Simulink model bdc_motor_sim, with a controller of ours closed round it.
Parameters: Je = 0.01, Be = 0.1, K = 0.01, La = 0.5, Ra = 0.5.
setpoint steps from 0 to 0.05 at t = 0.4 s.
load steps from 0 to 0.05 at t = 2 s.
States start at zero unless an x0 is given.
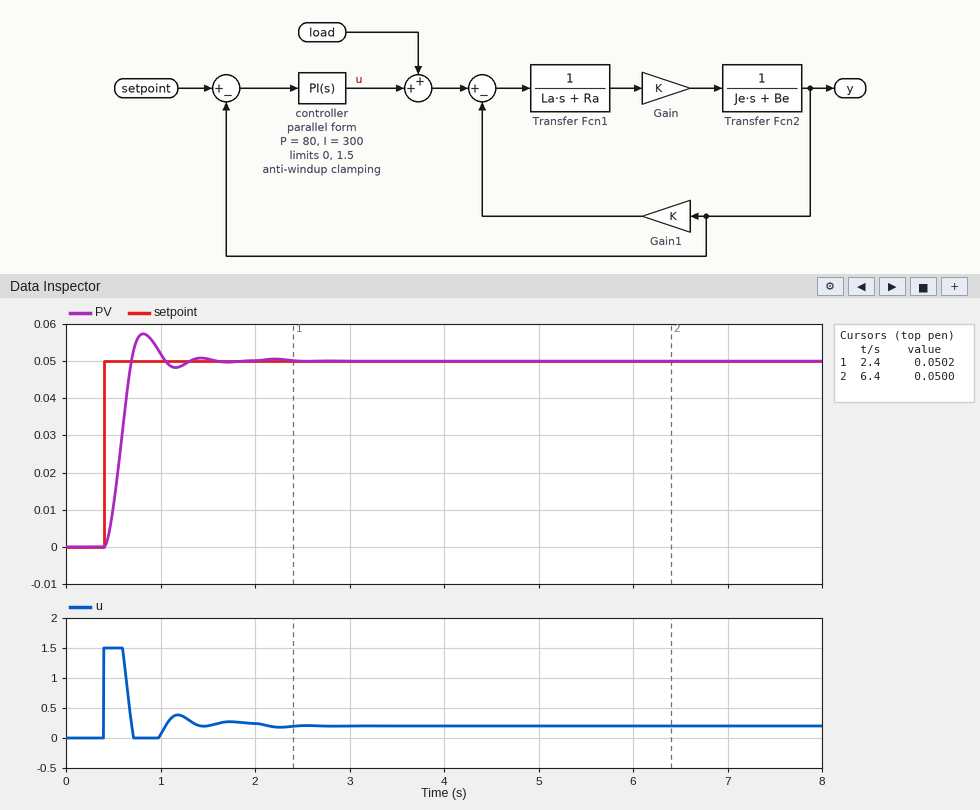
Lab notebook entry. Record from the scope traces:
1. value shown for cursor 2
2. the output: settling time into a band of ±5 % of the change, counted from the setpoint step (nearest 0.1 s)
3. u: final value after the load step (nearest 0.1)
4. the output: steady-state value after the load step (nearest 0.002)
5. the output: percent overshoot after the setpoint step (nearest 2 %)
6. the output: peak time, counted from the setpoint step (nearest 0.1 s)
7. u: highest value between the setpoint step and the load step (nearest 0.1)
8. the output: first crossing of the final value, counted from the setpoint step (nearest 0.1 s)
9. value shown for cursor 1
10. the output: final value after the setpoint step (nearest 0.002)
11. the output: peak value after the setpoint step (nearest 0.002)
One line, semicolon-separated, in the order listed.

0.0500; 0.6 s; 0.2; 0.050; 14 %; 0.4 s; 1.5; 0.3 s; 0.0502; 0.050; 0.058
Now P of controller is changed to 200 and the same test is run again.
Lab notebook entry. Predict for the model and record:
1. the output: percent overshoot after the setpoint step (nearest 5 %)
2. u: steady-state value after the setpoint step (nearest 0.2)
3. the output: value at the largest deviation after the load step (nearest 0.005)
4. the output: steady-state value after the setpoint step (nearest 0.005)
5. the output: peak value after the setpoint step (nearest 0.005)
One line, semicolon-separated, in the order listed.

20 %; 0.2; 0.050; 0.050; 0.060
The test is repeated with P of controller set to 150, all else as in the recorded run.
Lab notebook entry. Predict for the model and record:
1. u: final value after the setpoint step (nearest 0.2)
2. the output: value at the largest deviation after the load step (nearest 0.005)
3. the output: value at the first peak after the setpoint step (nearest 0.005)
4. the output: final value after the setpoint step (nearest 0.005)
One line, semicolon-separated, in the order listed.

0.2; 0.050; 0.060; 0.050
